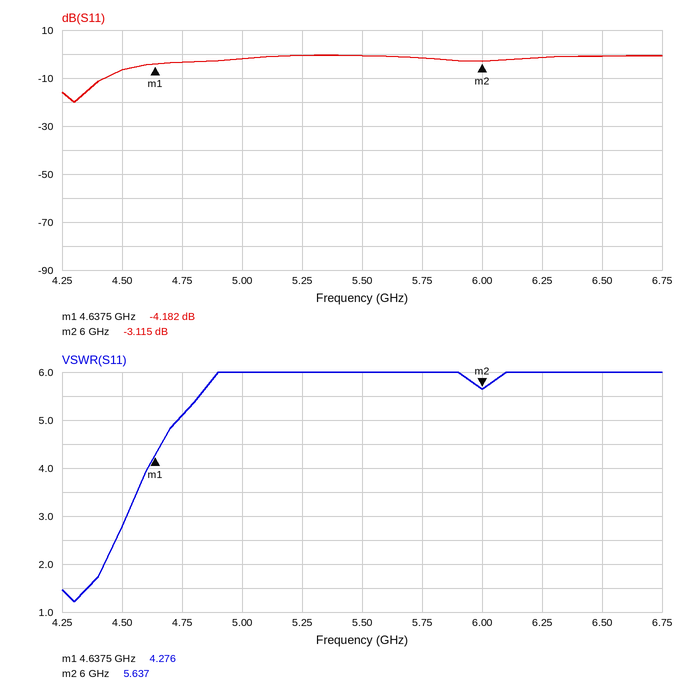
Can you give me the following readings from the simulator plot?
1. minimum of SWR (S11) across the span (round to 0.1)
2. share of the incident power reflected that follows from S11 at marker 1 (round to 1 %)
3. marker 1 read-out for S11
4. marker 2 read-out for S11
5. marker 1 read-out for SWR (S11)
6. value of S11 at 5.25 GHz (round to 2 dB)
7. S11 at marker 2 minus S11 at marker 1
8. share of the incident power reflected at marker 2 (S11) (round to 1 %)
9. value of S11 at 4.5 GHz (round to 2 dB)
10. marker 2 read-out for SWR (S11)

1.2
38 %
-4.182 dB
-3.115 dB
4.276
0 dB
1.067 dB
49 %
-6 dB
5.637
